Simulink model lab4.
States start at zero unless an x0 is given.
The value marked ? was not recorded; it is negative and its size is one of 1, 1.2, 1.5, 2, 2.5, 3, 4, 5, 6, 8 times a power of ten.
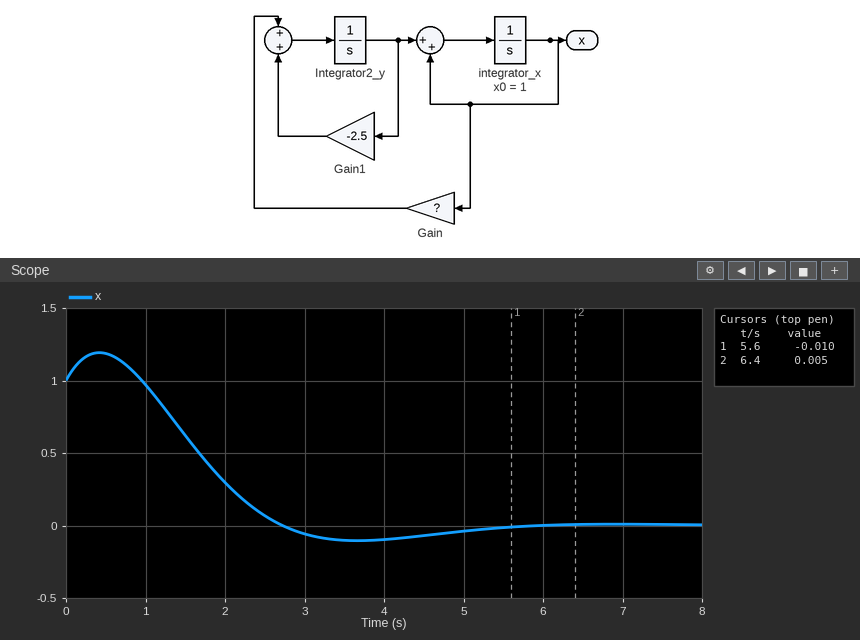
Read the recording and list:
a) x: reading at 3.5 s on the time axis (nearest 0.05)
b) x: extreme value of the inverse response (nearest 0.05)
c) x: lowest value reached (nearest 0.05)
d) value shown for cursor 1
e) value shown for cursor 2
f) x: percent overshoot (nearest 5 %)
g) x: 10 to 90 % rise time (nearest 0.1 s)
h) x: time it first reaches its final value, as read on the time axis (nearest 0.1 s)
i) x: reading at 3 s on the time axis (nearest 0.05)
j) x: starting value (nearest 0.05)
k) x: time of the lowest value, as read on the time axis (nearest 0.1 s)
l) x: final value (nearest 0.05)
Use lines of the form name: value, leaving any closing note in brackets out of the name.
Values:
x: reading at 3.5 s on the time axis: -0.10
x: extreme value of the inverse response: 1.20
x: lowest value reached: -0.10
value shown for cursor 1: -0.010
value shown for cursor 2: 0.005
x: percent overshoot: 10 %
x: 10 to 90 % rise time: 1.3 s
x: time it first reaches its final value, as read on the time axis: 2.7 s
x: reading at 3 s on the time axis: -0.05
x: starting value: 1.00
x: time of the lowest value, as read on the time axis: 3.7 s
x: final value: 0.00
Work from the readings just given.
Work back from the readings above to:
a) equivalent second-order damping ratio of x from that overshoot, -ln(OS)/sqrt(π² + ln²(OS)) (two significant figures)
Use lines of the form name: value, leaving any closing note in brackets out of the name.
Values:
equivalent second-order damping ratio of x from that overshoot, -ln(OS)/sqrt(π² + ln²(OS)): 0.59
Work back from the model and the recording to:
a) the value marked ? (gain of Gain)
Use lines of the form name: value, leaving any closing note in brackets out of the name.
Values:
the value marked ?: -4
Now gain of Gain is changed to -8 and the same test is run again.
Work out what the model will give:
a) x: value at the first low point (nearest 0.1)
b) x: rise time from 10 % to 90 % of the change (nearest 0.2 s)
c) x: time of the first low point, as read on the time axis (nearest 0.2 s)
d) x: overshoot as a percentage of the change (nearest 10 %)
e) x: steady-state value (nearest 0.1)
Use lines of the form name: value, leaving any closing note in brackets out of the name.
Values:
x: value at the first low point: -0.4
x: rise time from 10 % to 90 % of the change: 0.6 s
x: time of the first low point, as read on the time axis: 1.6 s
x: overshoot as a percentage of the change: 40 %
x: steady-state value: 0.0
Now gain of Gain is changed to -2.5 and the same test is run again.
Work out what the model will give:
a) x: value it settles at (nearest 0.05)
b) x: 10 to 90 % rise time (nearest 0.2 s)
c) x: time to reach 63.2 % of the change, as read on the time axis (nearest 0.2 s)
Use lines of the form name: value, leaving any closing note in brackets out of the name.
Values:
x: value it settles at: 1.65
x: 10 to 90 % rise time: 1.4 s
x: time to reach 63.2 % of the change, as read on the time axis: 0.6 s
